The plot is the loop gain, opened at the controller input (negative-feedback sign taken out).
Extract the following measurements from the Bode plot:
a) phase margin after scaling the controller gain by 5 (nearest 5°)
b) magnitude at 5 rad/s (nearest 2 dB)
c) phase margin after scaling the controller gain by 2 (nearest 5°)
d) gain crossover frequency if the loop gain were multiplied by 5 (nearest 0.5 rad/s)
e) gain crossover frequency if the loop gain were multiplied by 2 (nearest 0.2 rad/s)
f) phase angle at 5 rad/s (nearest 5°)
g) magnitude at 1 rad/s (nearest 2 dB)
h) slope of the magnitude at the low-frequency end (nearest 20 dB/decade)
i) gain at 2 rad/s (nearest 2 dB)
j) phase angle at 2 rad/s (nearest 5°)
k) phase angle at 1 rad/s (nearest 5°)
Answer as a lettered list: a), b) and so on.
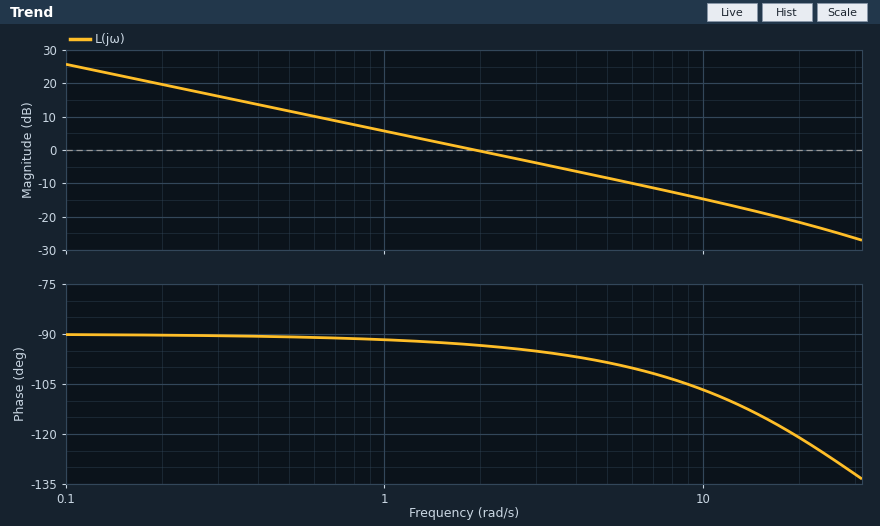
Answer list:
a) 75°
b) -8 dB
c) 85°
d) 9.5 rad/s
e) 3.8 rad/s
f) -100°
g) 6 dB
h) -20 dB/decade
i) 0 dB
j) -95°
k) -90°
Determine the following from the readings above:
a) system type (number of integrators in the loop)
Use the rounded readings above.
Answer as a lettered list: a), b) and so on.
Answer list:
a) 1
